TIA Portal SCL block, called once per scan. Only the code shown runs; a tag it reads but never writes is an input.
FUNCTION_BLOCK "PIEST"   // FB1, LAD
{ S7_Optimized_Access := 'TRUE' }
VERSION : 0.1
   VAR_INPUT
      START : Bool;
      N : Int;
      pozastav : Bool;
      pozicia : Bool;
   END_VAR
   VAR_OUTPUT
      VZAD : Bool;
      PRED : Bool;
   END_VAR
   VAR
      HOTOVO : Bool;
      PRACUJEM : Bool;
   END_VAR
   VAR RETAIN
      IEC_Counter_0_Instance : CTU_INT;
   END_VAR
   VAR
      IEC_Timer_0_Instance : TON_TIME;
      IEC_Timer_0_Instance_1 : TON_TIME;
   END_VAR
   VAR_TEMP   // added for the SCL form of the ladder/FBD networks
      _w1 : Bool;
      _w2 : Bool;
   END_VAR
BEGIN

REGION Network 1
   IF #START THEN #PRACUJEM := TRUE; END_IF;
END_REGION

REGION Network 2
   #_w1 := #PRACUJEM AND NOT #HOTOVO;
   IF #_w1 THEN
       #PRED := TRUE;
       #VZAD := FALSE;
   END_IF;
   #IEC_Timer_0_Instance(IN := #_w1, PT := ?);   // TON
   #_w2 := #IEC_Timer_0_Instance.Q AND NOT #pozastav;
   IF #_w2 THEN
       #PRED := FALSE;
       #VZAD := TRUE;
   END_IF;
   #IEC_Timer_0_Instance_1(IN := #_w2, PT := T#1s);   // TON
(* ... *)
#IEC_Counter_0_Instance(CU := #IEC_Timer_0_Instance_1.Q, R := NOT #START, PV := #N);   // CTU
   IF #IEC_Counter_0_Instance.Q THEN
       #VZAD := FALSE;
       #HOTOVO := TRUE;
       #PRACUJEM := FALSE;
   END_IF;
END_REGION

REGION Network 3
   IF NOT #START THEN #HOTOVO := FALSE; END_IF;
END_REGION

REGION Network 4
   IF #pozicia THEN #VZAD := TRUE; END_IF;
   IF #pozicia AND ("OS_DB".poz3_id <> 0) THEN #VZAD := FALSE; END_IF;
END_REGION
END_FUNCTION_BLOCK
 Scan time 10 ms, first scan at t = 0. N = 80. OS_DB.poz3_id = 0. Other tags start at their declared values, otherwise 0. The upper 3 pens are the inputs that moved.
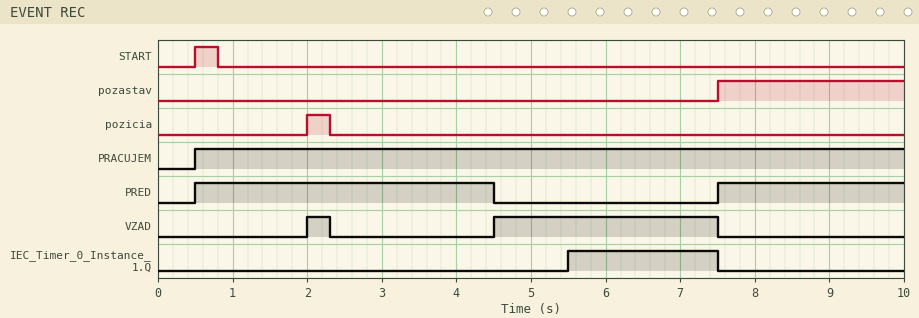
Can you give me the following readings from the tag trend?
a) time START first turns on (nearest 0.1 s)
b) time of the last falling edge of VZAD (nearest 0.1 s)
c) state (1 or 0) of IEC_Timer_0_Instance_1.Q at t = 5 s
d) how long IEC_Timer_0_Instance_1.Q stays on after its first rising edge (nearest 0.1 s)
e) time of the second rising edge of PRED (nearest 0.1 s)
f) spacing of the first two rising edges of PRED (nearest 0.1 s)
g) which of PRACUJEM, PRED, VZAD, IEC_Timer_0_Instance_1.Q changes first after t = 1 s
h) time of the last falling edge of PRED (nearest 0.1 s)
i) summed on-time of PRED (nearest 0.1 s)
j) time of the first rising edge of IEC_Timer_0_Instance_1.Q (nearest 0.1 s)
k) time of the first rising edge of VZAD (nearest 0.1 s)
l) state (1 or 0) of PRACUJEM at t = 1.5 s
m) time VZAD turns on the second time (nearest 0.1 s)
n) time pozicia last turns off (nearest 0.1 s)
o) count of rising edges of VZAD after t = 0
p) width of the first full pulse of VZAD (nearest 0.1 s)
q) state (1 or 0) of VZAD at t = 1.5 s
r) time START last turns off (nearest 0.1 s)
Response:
0.5 s
7.5 s
0
2.0 s
7.5 s
7.0 s
VZAD
4.5 s
6.5 s
5.5 s
2.0 s
1
4.5 s
2.3 s
2
0.3 s
0
0.8 s
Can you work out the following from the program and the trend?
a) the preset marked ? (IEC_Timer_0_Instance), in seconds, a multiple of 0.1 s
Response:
4.0 s
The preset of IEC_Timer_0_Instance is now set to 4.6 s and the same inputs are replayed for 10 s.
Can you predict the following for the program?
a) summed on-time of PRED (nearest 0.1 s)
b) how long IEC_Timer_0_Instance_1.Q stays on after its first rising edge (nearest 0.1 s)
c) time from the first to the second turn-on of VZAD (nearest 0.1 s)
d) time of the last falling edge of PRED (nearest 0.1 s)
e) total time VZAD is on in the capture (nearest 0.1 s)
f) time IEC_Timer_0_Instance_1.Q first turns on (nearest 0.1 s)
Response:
7.1 s
1.4 s
3.1 s
5.1 s
2.7 s
6.1 s
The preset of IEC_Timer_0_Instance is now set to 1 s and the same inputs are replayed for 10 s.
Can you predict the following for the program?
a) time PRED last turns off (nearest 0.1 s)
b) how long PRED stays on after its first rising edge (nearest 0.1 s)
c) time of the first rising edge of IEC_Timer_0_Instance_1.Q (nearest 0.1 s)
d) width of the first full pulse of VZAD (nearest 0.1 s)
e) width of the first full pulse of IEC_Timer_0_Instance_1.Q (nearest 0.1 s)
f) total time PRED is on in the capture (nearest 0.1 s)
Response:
1.5 s
1.0 s
2.5 s
6.0 s
5.0 s
3.5 s
